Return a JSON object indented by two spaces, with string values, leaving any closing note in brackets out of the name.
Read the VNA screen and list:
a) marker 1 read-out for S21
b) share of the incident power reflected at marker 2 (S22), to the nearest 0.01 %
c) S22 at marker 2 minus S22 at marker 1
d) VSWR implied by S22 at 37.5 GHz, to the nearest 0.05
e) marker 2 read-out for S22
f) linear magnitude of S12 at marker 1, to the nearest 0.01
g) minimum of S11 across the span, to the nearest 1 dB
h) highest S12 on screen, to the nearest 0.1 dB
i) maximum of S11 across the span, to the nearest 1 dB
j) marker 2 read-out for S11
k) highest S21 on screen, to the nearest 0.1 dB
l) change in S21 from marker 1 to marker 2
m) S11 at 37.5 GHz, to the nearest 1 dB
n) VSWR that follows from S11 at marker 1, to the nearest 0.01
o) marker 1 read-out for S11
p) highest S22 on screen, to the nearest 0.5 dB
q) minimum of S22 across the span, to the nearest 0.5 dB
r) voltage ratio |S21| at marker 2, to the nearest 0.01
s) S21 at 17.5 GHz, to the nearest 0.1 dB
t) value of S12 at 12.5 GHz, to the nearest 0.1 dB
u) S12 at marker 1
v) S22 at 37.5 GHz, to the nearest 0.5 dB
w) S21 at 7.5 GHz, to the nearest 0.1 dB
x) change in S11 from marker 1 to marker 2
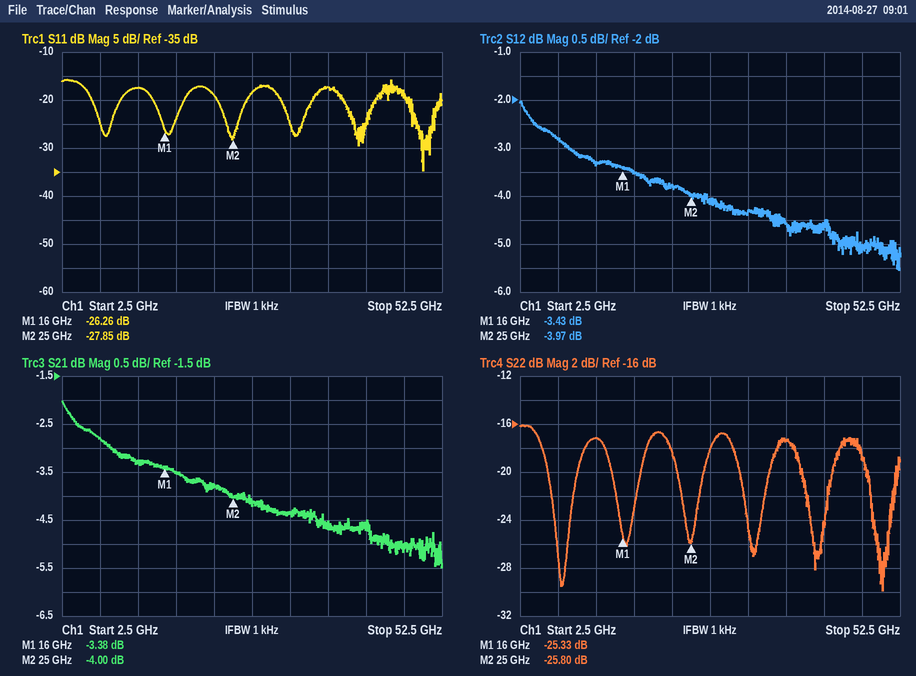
{
  "marker 1 read-out for S21": "-3.38 dB",
  "share of the incident power reflected at marker 2 (S22), to the nearest 0.01 %": "0.26 %",
  "S22 at marker 2 minus S22 at marker 1": "-0.47 dB",
  "VSWR implied by S22 at 37.5 GHz, to the nearest 0.05": "1.30",
  "marker 2 read-out for S22": "-25.80 dB",
  "linear magnitude of S12 at marker 1, to the nearest 0.01": "0.67",
  "minimum of S11 across the span, to the nearest 1 dB": "-35 dB",
  "highest S12 on screen, to the nearest 0.1 dB": "-2.0 dB",
  "maximum of S11 across the span, to the nearest 1 dB": "-16 dB",
  "marker 2 read-out for S11": "-27.85 dB",
  "highest S21 on screen, to the nearest 0.1 dB": "-2.0 dB",
  "change in S21 from marker 1 to marker 2": "-0.62 dB",
  "S11 at 37.5 GHz, to the nearest 1 dB": "-17 dB",
  "VSWR that follows from S11 at marker 1, to the nearest 0.01": "1.10",
  "marker 1 read-out for S11": "-26.26 dB",
  "highest S22 on screen, to the nearest 0.5 dB": "-16.0 dB",
  "minimum of S22 across the span, to the nearest 0.5 dB": "-30.0 dB",
  "voltage ratio |S21| at marker 2, to the nearest 0.01": "0.63",
  "S21 at 17.5 GHz, to the nearest 0.1 dB": "-3.5 dB",
  "value of S12 at 12.5 GHz, to the nearest 0.1 dB": "-3.3 dB",
  "S12 at marker 1": "-3.43 dB",
  "S22 at 37.5 GHz, to the nearest 0.5 dB": "-17.5 dB",
  "S21 at 7.5 GHz, to the nearest 0.1 dB": "-2.8 dB",
  "change in S11 from marker 1 to marker 2": "-1.59 dB"
}
